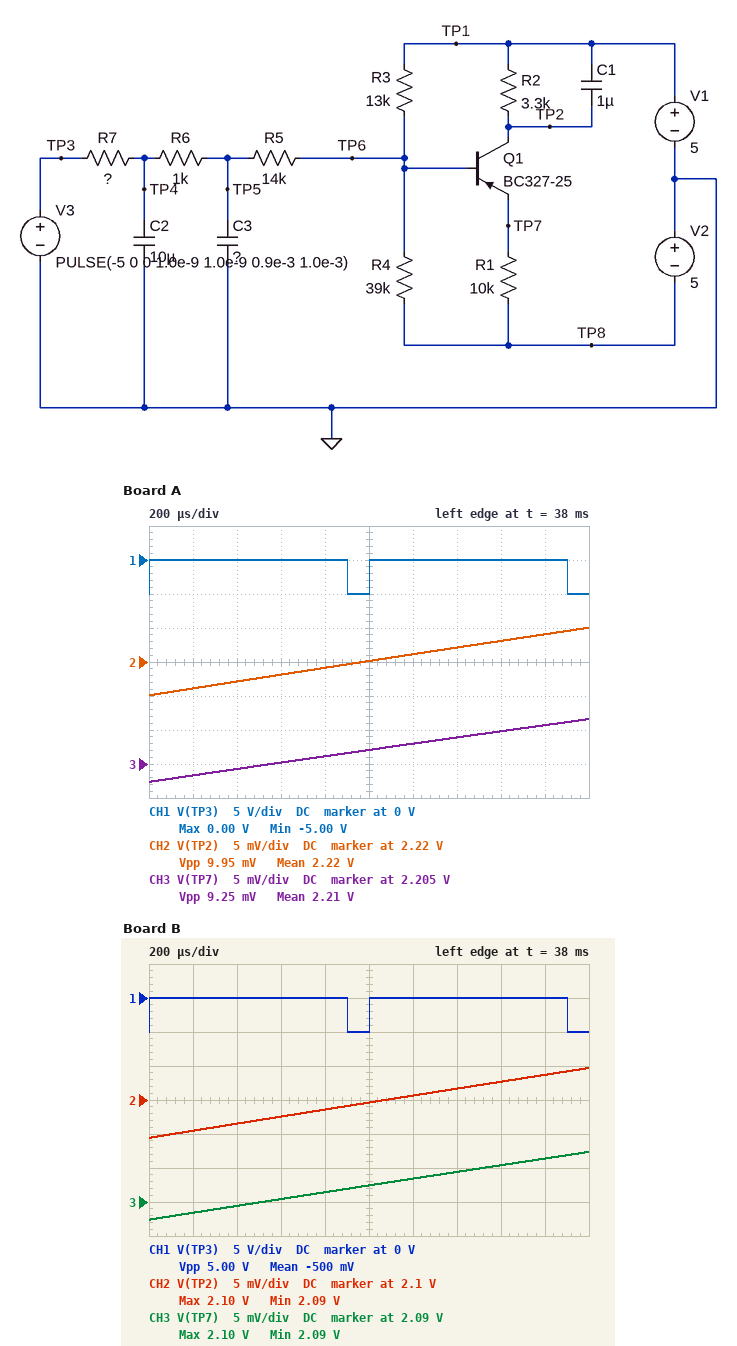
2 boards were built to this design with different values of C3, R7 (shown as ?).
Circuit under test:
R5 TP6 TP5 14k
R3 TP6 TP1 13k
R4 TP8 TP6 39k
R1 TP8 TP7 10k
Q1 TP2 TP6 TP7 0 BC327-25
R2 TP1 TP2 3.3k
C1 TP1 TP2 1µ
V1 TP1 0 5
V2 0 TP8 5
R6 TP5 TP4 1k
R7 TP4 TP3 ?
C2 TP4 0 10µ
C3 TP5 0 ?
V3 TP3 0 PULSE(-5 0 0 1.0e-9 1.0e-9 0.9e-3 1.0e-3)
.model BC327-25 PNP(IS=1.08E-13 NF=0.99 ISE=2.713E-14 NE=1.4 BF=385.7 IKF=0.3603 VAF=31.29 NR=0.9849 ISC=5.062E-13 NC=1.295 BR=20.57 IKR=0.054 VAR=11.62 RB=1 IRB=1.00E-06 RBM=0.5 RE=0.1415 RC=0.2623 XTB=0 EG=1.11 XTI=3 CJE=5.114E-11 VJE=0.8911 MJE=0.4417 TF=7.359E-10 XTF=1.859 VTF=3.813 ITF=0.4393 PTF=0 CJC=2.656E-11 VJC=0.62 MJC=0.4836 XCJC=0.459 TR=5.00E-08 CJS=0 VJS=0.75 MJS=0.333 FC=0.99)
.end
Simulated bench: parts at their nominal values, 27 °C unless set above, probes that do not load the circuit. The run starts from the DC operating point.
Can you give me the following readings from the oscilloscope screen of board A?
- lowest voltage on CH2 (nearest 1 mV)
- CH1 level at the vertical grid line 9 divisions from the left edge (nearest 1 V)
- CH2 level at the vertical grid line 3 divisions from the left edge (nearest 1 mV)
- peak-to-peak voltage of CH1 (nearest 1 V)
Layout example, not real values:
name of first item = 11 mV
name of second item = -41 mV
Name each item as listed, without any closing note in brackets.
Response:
lowest voltage on CH2 = 2.215 V
CH1 level at the vertical grid line 9 divisions from the left edge = 0 V
CH2 level at the vertical grid line 3 divisions from the left edge = 2.218 V
peak-to-peak voltage of CH1 = 5 V
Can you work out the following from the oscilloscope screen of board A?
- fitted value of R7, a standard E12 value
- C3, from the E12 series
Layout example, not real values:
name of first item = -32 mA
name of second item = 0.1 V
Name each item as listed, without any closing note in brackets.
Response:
fitted value of R7, a standard E12 value = 2.2 kΩ
C3, from the E12 series = 5.6 µF
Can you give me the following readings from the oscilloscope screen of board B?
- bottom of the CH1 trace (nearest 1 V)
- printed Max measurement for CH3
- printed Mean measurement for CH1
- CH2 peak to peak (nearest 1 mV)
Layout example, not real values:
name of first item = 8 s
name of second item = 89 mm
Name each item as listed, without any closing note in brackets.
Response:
bottom of the CH1 trace = -5 V
printed Max measurement for CH3 = 2.10 V
printed Mean measurement for CH1 = -500 mV
CH2 peak to peak = 10 mV
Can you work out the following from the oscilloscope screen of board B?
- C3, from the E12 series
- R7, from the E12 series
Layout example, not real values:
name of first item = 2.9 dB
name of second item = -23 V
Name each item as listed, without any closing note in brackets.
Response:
C3, from the E12 series = 33 µF
R7, from the E12 series = 560 Ω
